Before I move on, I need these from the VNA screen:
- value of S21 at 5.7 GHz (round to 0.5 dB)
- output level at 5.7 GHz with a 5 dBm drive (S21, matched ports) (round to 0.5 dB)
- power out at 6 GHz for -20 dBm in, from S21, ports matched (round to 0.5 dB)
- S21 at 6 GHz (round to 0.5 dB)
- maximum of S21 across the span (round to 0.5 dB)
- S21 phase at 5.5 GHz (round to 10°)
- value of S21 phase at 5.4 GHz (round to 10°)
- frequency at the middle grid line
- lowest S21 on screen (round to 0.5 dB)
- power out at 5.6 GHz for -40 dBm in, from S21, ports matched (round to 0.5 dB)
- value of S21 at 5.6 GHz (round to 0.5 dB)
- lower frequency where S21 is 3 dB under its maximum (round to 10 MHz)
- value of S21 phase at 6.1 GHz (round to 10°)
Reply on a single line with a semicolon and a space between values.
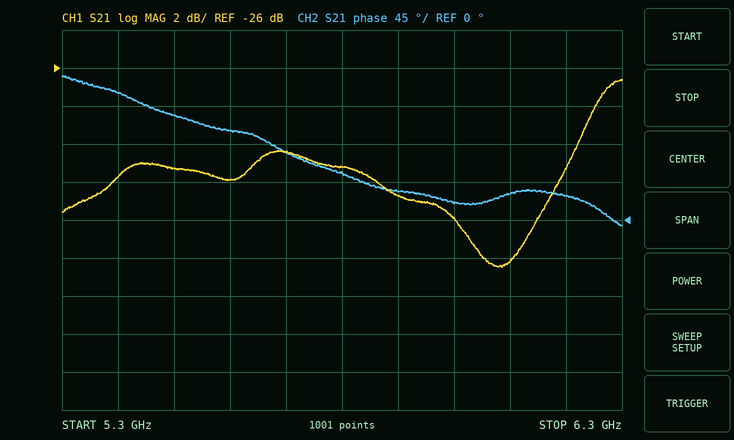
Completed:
-30.5 dB; -25.5 dBm; -54.0 dBm; -34.0 dB; -26.5 dB; 120°; 150°; 5.8 GHz; -36.5 dB; -72.0 dBm; -32.0 dB; 6.23 GHz; 30°
